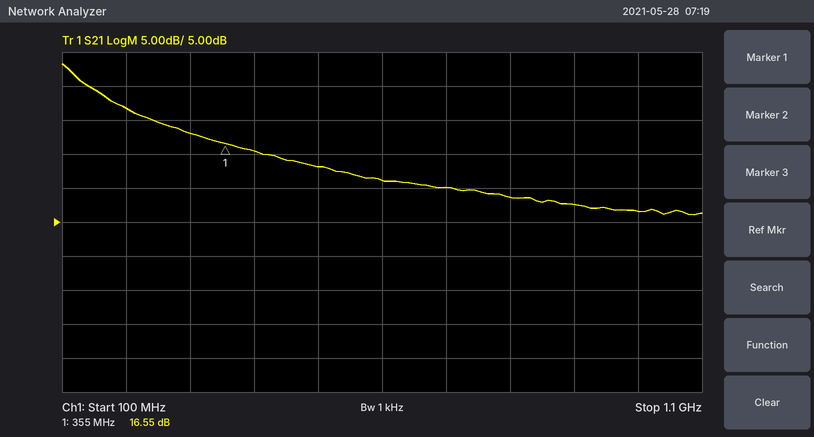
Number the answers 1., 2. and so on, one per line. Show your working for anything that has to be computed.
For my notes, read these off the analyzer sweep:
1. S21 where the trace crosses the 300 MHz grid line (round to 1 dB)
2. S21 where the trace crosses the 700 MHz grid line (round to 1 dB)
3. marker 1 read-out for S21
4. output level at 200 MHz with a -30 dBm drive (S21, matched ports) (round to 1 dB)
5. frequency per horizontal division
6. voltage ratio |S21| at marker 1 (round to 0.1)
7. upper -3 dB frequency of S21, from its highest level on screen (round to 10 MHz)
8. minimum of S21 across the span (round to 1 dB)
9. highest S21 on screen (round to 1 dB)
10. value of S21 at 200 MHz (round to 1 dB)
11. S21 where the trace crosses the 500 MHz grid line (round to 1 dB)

1. 18 dB
2. 10 dB
3. 16.55 dB
4. -30 dBm + (22 dB) = -8 dBm
5. 100 MHz
6. 10^(16.55/20) ≈ 6.7
7. 140 MHz
8. 6 dB
9. 28 dB
10. 22 dB
11. 13 dB
